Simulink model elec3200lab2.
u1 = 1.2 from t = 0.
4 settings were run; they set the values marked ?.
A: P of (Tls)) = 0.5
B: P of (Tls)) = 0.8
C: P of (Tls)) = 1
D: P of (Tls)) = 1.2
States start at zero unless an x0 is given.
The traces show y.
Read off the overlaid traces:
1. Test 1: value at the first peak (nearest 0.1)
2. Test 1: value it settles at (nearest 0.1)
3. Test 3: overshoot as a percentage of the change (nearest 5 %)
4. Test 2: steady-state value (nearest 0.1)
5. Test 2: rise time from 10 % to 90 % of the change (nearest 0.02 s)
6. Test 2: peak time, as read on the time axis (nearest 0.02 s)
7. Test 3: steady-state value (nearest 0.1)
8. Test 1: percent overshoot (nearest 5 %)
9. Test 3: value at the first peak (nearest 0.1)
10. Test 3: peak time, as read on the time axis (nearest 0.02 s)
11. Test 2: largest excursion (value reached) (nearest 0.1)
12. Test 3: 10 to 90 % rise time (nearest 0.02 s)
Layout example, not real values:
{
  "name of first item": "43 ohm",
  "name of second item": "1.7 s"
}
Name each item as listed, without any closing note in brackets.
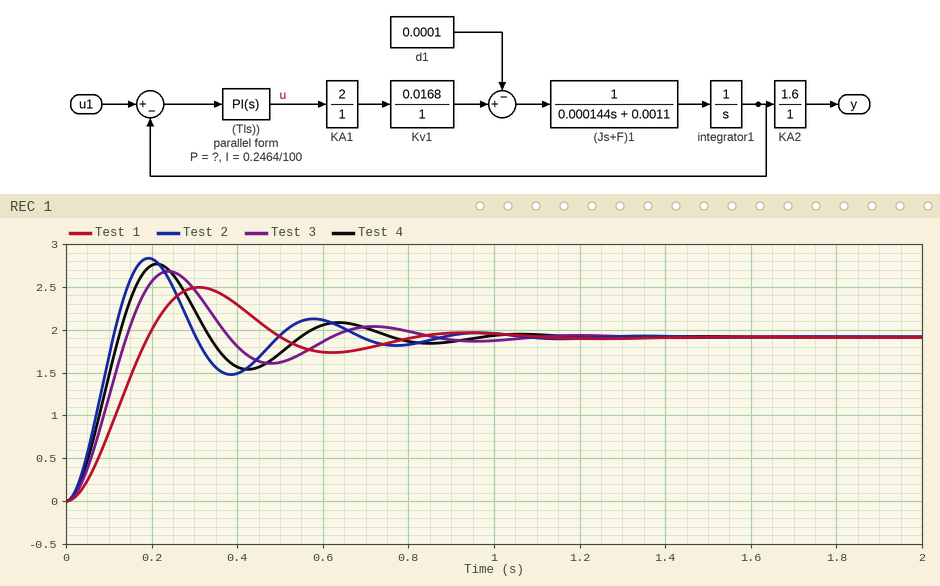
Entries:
{
  "Test 1: value at the first peak": "2.5",
  "Test 1: value it settles at": "1.9",
  "Test 3: overshoot as a percentage of the change": "40 %",
  "Test 2: steady-state value": "1.9",
  "Test 2: rise time from 10 % to 90 % of the change": "0.08 s",
  "Test 2: peak time, as read on the time axis": "0.20 s",
  "Test 3: steady-state value": "1.9",
  "Test 1: percent overshoot": "30 %",
  "Test 3: value at the first peak": "2.7",
  "Test 3: peak time, as read on the time axis": "0.24 s",
  "Test 2: largest excursion (value reached)": "2.8",
  "Test 3: 10 to 90 % rise time": "0.10 s"
}
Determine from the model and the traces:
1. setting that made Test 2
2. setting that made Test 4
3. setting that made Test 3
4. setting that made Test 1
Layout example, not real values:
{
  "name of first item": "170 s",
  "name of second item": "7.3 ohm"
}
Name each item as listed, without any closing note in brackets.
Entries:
{
  "setting that made Test 2": "D",
  "setting that made Test 4": "C",
  "setting that made Test 3": "B",
  "setting that made Test 1": "A"
}
